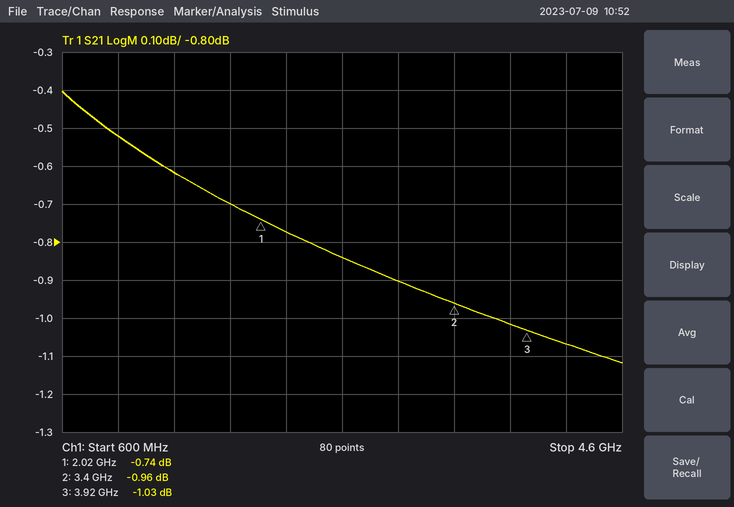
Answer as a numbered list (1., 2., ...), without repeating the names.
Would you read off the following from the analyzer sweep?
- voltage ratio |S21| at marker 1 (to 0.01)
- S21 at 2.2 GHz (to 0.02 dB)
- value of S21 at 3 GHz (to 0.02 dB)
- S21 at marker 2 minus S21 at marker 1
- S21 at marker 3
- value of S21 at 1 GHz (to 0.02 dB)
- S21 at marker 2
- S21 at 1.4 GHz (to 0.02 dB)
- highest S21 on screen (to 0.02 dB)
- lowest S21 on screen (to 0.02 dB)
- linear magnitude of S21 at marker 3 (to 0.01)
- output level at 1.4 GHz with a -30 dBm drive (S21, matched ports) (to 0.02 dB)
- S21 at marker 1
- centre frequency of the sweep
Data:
1. 0.92
2. -0.78 dB
3. -0.90 dB
4. -0.22 dB
5. -1.03 dB
6. -0.52 dB
7. -0.96 dB
8. -0.62 dB
9. -0.40 dB
10. -1.12 dB
11. 0.89
12. -30.62 dBm
13. -0.74 dB
14. 2.6 GHz
